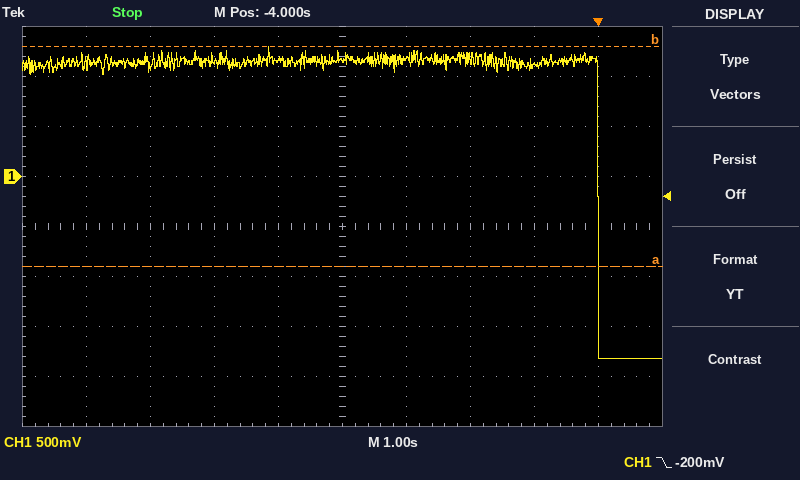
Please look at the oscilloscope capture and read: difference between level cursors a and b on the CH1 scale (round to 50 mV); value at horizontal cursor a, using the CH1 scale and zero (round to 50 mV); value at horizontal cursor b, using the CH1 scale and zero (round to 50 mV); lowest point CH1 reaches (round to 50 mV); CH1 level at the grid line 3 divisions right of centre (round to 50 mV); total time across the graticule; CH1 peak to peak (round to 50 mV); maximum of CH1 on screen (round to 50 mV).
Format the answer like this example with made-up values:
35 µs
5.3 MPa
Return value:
2.20 V
-900 mV
1.30 V
-1.80 V
1.10 V
10 s
3.10 V
1.30 V
